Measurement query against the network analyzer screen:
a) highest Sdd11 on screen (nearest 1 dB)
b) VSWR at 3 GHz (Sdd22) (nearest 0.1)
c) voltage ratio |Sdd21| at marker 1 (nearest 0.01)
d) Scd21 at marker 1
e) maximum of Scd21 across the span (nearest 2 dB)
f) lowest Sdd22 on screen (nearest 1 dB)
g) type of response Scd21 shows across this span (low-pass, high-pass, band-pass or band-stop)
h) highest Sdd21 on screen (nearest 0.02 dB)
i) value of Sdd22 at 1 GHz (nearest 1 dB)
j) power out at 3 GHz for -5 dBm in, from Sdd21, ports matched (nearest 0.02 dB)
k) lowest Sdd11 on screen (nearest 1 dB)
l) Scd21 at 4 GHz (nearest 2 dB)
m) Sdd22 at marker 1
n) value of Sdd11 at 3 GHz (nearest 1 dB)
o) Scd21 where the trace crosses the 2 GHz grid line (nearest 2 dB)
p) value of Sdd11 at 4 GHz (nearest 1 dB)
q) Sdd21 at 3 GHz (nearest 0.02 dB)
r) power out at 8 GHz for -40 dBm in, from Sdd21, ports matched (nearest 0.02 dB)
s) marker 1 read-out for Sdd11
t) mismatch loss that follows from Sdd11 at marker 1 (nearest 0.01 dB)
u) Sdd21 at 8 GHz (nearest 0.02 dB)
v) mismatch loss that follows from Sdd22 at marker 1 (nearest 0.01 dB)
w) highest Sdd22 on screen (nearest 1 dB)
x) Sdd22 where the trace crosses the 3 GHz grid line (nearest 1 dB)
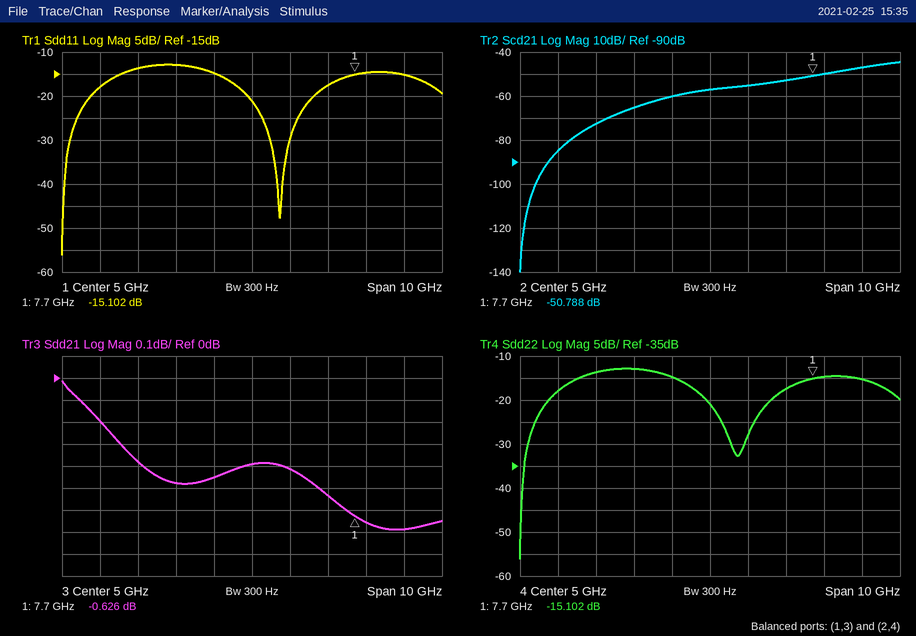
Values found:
-13 dB
1.6
0.93
-50.788 dB
-44 dB
-56 dB
high-pass
-0.02 dB
-18 dB
-5.48 dBm
-56 dB
-60 dB
-15.102 dB
-13 dB
-72 dB
-15 dB
-0.48 dB
-40.66 dBm
-15.102 dB
0.14 dB
-0.66 dB
0.14 dB
-13 dB
-13 dB
